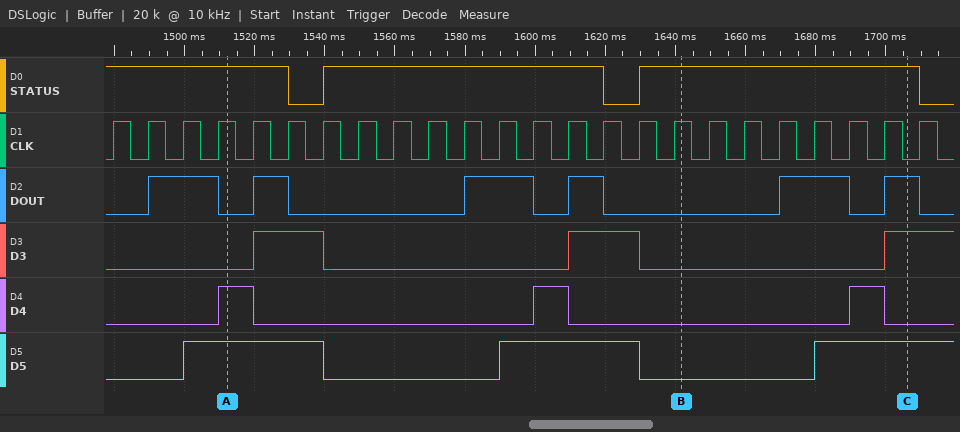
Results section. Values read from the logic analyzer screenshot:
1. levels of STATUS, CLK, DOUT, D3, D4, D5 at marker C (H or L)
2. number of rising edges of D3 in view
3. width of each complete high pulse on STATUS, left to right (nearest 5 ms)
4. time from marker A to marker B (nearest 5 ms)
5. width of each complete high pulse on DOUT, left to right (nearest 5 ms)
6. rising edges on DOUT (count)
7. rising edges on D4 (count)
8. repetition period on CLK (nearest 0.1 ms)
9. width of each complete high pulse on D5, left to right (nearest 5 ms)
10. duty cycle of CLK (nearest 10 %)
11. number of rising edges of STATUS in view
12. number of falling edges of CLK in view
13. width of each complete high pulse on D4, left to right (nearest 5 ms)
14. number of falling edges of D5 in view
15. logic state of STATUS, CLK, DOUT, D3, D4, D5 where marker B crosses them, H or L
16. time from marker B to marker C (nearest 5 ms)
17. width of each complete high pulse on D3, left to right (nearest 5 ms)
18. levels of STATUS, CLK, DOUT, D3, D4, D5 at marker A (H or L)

STATUS=H, CLK=L, DOUT=H, D3=H, D4=L, D5=H
3
80 ms, 80 ms
130 ms
20 ms, 10 ms, 20 ms, 10 ms, 20 ms, 10 ms
6
3
10 ms
40 ms, 40 ms
50 %
2
24
10 ms, 10 ms, 10 ms
2
STATUS=H, CLK=H, DOUT=L, D3=L, D4=L, D5=L
65 ms
20 ms, 20 ms
STATUS=H, CLK=H, DOUT=L, D3=L, D4=H, D5=H
